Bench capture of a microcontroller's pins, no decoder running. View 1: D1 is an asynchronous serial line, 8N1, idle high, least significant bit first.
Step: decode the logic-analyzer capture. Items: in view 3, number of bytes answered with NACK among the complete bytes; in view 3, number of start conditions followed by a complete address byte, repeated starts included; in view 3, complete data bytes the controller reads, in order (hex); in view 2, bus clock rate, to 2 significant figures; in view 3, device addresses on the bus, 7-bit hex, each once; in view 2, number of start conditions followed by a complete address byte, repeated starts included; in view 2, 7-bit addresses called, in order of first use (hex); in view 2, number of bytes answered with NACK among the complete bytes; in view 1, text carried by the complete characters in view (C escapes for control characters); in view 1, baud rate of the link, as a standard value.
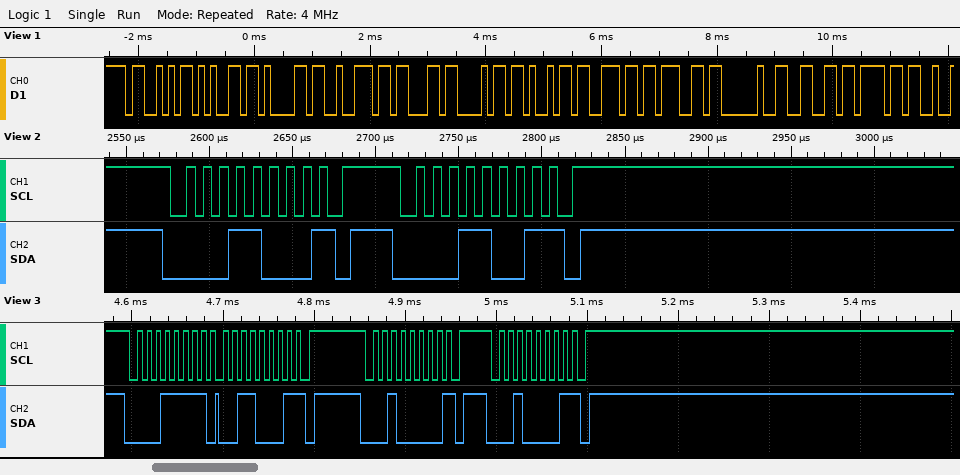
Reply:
3
3
31
100 kHz
0x0F 0x10
2
0x0C
2
"Searching fo"
9600 baud
